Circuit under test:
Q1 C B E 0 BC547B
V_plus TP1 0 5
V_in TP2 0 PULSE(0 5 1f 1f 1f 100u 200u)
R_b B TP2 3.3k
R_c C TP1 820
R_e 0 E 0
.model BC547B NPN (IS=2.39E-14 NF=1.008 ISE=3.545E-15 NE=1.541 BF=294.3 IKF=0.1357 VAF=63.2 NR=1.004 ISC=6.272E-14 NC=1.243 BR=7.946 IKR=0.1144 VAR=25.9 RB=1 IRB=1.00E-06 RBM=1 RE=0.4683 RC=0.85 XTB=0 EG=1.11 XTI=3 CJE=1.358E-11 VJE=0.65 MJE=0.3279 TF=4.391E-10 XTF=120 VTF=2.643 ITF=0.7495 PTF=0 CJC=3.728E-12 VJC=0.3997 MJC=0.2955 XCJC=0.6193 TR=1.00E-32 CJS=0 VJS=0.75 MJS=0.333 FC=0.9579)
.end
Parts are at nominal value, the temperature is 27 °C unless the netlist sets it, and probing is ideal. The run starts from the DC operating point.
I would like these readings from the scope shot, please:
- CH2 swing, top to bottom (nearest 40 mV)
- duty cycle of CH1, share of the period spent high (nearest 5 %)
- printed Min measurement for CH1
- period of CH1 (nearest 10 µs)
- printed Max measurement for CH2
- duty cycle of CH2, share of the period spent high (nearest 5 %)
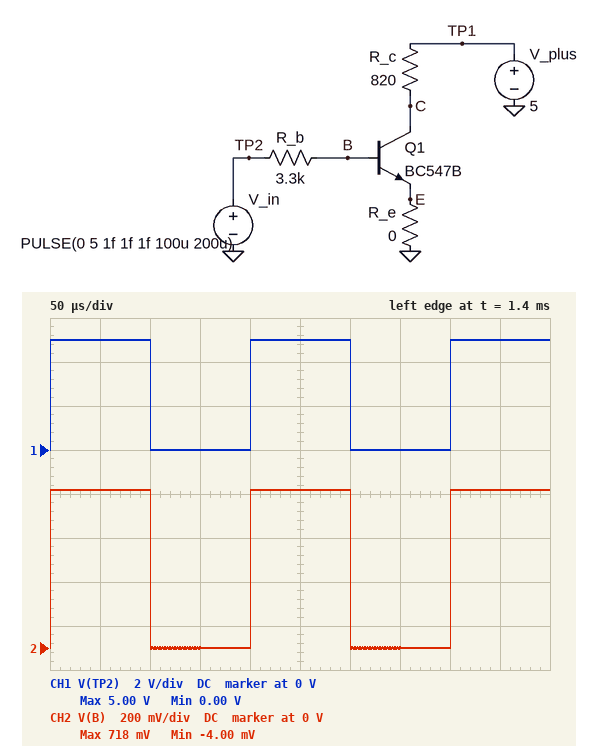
720 mV
50 %
0.00 V
200 µs
718 mV
50 %
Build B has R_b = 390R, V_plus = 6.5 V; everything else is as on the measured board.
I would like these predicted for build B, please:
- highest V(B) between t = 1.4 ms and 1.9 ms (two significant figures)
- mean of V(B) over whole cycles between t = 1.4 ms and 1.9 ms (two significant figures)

780 mV
390 mV
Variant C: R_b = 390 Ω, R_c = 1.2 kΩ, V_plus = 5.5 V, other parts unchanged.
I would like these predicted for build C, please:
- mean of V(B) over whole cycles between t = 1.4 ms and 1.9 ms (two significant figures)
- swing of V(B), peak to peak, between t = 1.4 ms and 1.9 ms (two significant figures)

390 mV
780 mV
